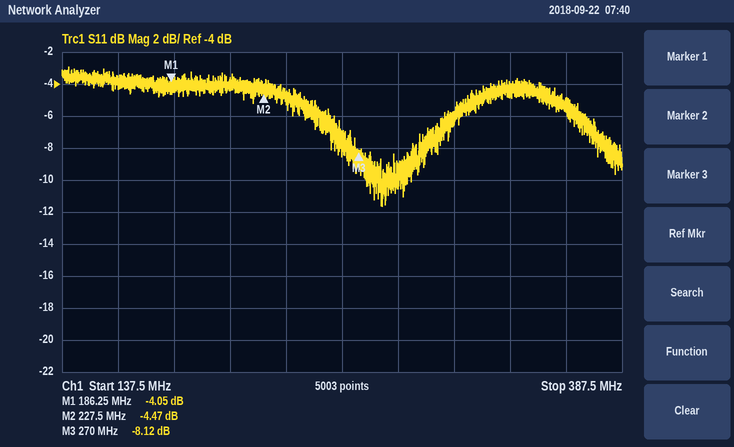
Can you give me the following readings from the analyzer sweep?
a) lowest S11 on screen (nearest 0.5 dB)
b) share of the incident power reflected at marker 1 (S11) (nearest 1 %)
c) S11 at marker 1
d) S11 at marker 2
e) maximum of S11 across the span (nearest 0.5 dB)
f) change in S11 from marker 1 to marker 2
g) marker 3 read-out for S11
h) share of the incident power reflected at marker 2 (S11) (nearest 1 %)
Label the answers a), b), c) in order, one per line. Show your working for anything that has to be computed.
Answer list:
a) -11.5 dB
b) 10^(-4.05/10) ≈ 39 %
c) -4.05 dB
d) -4.47 dB
e) -3.0 dB
f) -4.47 − (-4.05) = -0.42 dB
g) -8.12 dB
h) 10^(-4.47/10) ≈ 36 %
